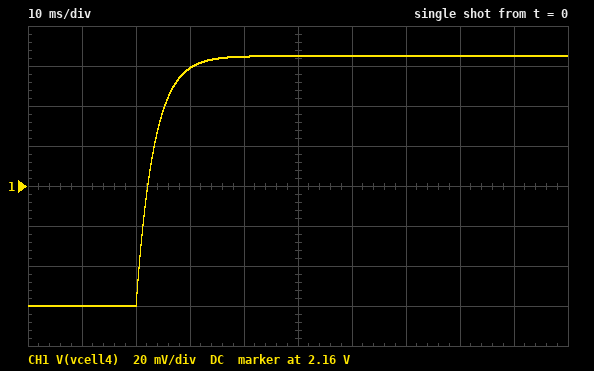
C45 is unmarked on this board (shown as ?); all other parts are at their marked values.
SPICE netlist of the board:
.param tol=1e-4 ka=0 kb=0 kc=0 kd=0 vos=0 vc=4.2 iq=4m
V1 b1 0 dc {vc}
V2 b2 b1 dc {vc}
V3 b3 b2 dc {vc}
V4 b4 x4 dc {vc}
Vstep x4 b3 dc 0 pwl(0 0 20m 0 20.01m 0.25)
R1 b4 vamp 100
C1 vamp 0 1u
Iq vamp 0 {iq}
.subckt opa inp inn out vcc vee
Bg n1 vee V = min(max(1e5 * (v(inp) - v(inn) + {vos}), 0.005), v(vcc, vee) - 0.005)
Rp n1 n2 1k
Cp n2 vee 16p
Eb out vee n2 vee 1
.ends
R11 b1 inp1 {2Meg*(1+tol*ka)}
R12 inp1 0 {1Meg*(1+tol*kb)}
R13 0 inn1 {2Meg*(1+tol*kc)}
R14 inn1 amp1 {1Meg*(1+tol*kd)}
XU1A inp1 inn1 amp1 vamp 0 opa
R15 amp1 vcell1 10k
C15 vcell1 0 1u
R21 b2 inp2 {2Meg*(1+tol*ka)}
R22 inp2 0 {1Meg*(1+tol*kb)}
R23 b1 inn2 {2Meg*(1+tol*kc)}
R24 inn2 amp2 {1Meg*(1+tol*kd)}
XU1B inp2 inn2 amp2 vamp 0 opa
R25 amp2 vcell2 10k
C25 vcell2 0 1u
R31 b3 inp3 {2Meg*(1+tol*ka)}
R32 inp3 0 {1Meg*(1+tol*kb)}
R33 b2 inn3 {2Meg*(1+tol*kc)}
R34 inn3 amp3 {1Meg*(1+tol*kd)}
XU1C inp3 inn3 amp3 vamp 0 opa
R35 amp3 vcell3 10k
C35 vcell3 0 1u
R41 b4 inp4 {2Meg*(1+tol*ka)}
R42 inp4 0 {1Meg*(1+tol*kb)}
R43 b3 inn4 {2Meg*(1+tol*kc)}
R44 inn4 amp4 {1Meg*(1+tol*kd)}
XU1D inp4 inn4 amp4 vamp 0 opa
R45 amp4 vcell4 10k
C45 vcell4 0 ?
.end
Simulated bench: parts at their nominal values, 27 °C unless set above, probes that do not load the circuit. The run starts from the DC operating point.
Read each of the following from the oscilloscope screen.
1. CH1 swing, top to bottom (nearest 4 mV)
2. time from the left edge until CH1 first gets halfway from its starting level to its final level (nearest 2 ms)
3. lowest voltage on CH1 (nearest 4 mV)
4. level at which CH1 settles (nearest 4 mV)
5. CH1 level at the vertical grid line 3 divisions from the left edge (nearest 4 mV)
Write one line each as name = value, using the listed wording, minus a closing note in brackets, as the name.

CH1 swing, top to bottom = 124 mV
time from the left edge until CH1 first gets halfway from its starting level to its final level = 22 ms
lowest voltage on CH1 = 2.100 V
level at which CH1 settles = 2.224 V
CH1 level at the vertical grid line 3 divisions from the left edge = 2.220 V
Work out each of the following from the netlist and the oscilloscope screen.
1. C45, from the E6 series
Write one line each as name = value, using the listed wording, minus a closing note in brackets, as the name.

C45, from the E6 series = 330 nF
